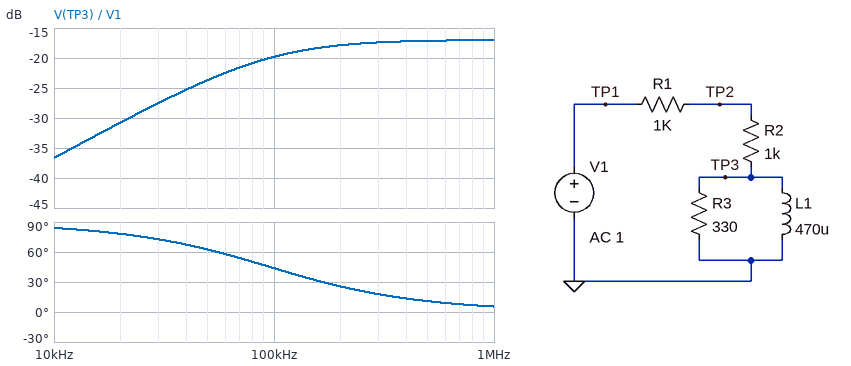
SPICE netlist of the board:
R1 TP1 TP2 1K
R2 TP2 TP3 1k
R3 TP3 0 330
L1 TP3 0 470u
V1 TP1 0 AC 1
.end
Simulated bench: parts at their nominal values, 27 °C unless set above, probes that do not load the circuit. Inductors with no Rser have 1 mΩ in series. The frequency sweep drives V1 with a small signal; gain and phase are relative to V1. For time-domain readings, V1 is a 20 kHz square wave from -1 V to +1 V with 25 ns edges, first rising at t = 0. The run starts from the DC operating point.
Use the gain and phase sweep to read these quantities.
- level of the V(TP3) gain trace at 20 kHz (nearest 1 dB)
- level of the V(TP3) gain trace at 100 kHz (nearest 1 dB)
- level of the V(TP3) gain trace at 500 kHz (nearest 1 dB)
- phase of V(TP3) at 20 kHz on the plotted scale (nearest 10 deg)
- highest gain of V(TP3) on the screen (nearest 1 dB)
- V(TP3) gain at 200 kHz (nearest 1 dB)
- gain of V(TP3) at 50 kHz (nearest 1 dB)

-31 dB
-20 dB
-17 dB
80 deg
-17 dB
-18 dB
-24 dB
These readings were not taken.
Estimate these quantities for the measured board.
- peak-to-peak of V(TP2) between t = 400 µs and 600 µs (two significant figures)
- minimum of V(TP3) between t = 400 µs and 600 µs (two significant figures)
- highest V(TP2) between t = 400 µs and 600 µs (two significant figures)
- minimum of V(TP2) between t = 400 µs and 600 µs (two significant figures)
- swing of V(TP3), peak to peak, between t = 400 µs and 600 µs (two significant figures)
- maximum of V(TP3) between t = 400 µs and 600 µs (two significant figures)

1.3 V
-280 mV
640 mV
-640 mV
560 mV
280 mV
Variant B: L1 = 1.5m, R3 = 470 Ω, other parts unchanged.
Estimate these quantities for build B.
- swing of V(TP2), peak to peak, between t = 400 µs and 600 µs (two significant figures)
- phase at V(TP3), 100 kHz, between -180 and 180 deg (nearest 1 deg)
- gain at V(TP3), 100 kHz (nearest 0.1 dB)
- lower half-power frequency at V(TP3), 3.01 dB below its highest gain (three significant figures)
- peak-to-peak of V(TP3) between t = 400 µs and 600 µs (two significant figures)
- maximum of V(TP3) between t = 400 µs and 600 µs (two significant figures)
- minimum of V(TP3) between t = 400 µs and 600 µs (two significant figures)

1.4 V
22 deg
-15.1 dB
40.4 kHz
760 mV
380 mV
-380 mV
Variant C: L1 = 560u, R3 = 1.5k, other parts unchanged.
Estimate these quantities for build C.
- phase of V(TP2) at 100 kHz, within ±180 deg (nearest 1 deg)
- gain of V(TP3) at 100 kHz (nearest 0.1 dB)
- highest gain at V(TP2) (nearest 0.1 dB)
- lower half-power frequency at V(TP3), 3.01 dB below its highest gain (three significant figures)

8 deg
-15.8 dB
-2.9 dB
244 kHz
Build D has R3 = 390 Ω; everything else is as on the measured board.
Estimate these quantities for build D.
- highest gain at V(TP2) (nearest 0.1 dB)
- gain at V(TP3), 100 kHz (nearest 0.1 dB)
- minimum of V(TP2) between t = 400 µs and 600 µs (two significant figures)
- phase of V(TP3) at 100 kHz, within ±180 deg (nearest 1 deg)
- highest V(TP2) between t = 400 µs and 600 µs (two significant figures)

-4.7 dB
-19.2 dB
-660 mV
48 deg
660 mV
